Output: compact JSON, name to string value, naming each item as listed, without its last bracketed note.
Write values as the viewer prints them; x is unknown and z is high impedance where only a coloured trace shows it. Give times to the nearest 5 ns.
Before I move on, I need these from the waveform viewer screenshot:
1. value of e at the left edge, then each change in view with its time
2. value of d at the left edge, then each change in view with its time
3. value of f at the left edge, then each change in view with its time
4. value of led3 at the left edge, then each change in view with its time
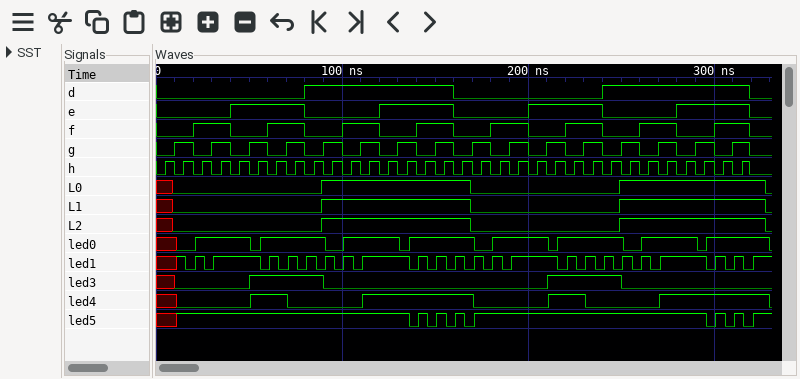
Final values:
{"value of e at the left edge, then each change in view with its time": "0, 1 at 40 ns, 0 at 80 ns, 1 at 120 ns, 0 at 160 ns, 1 at 200 ns, 0 at 240 ns, 1 at 280 ns, 0 at 320 ns", "value of d at the left edge, then each change in view with its time": "0, 1 at 80 ns, 0 at 160 ns, 1 at 240 ns, 0 at 320 ns", "value of f at the left edge, then each change in view with its time": "0, 1 at 20 ns, 0 at 40 ns, 1 at 60 ns, 0 at 80 ns, 1 at 100 ns, 0 at 120 ns, 1 at 140 ns, 0 at 160 ns, 1 at 180 ns, 0 at 200 ns, 1 at 220 ns, 0 at 240 ns, 1 at 260 ns, 0 at 280 ns, 1 at 300 ns, 0 at 320 ns", "value of led3 at the left edge, then each change in view with its time": "x, 0 at 10 ns, 1 at 50 ns, 0 at 90 ns, 1 at 210 ns, 0 at 250 ns"}
